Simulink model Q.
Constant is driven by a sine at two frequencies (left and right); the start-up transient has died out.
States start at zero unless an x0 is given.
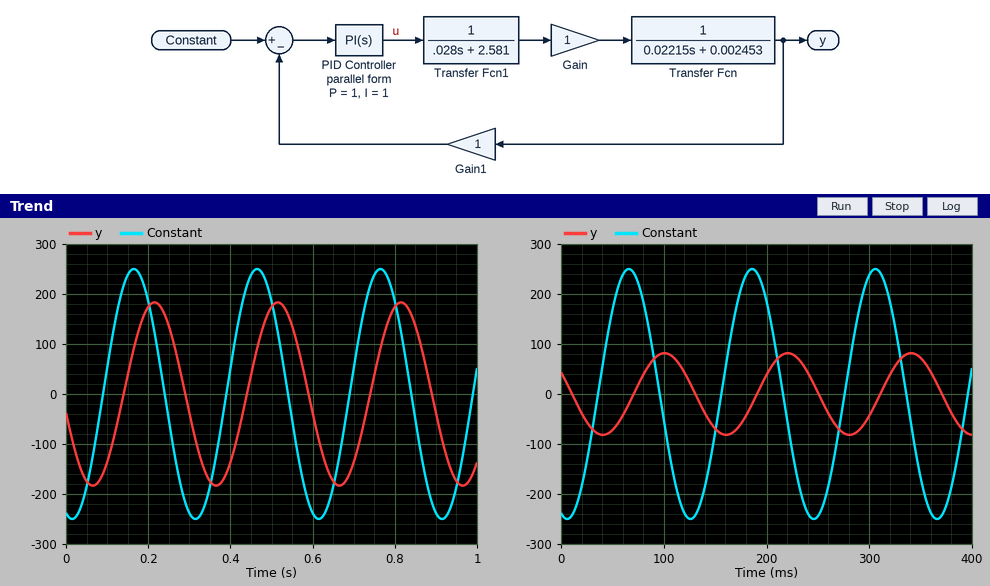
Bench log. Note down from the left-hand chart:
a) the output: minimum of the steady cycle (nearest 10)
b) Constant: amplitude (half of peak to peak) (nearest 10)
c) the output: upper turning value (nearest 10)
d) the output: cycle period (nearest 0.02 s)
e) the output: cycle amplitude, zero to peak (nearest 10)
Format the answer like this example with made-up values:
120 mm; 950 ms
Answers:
-180; 250; 180; 0.30 s; 180
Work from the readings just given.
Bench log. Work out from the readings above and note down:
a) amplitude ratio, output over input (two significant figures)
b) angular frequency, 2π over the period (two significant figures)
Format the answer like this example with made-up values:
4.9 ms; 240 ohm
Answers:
0.72; 21 rad/s
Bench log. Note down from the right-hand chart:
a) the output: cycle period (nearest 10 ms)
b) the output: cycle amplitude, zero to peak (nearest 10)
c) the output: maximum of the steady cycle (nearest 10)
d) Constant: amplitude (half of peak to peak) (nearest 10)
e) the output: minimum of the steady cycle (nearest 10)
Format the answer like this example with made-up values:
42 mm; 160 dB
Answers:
120 ms; 80; 80; 250; -80
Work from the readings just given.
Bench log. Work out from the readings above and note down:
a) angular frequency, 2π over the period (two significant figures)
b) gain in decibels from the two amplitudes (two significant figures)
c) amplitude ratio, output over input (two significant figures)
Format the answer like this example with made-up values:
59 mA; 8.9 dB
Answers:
0.052 rad/ms; -9.9 dB; 0.32
